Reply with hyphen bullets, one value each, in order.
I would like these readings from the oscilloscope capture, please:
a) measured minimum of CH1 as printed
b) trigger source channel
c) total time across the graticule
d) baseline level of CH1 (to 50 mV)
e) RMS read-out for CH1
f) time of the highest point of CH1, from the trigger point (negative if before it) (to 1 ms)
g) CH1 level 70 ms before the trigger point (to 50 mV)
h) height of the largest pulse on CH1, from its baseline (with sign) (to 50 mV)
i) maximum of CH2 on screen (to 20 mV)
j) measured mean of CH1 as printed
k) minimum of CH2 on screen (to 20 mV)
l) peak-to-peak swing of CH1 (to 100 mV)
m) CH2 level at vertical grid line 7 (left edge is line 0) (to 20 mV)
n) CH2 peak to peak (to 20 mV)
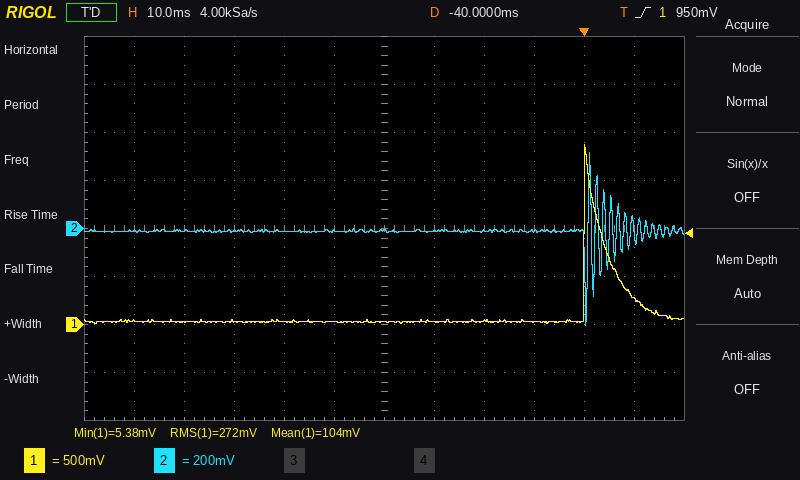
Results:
- 5.38 mV
- CH1
- 120 ms
- 50 mV
- 272 mV
- 0 ms
- 50 mV
- +1.85 V
- 320 mV
- 104 mV
- -400 mV
- 1.90 V
- 0 mV
- 720 mV
